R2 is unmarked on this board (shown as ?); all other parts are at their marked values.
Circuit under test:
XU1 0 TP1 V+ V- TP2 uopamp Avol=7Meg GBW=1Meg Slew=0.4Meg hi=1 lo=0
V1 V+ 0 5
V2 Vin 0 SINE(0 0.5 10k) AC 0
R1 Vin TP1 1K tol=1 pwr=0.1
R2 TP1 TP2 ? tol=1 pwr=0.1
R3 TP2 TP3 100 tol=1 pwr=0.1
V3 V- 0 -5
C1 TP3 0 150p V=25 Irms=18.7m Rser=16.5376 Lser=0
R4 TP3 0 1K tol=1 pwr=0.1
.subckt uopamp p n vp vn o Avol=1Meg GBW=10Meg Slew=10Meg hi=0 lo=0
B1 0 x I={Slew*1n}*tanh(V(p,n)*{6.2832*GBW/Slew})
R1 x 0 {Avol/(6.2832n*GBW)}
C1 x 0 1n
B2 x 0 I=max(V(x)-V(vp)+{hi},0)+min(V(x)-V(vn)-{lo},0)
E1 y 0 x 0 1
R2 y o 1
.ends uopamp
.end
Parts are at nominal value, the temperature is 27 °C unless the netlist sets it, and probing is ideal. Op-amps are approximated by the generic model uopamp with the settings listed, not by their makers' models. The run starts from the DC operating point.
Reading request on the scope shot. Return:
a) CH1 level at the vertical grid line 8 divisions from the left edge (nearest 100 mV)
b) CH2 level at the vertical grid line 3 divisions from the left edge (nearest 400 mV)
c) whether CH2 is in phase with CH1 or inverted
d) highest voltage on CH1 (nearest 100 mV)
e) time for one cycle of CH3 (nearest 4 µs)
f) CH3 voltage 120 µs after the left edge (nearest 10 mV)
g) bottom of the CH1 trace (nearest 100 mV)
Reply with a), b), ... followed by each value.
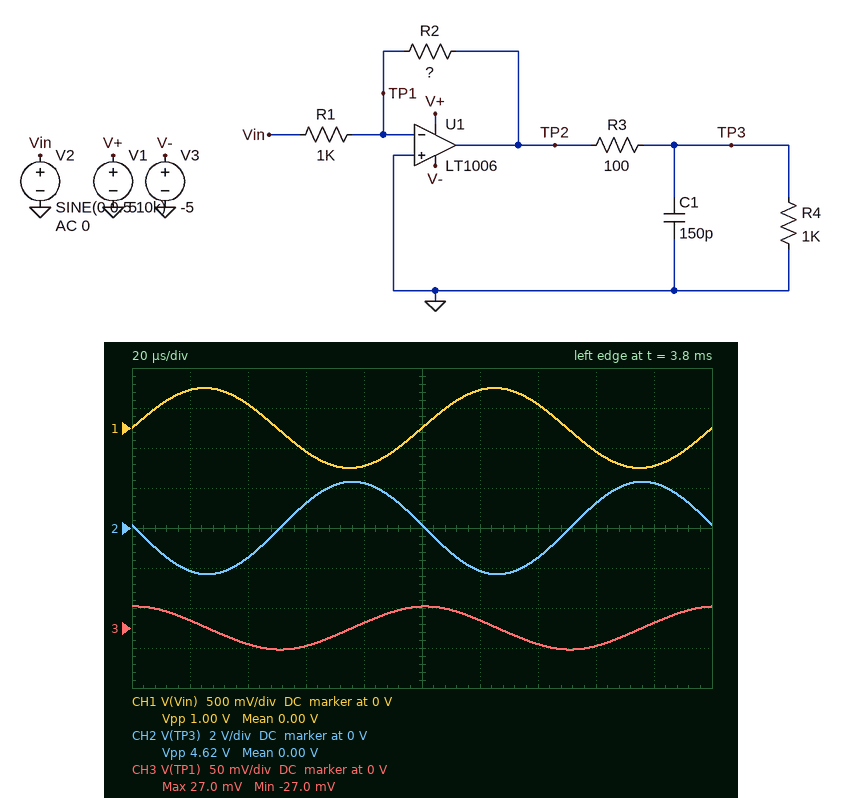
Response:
a) -300 mV
b) 1.2 V
c) inverted
d) 500 mV
e) 100 µs
f) 10 mV
g) -500 mV
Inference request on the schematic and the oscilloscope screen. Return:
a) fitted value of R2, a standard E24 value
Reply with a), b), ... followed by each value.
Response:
a) 5.1 kΩ
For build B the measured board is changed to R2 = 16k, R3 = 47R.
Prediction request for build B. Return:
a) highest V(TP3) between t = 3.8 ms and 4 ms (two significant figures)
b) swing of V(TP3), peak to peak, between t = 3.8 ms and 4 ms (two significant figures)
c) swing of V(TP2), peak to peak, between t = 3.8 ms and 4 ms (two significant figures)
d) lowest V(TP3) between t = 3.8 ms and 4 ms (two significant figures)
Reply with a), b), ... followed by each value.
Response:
a) 3.8 V
b) 8.6 V
c) 9.0 V
d) -4.8 V
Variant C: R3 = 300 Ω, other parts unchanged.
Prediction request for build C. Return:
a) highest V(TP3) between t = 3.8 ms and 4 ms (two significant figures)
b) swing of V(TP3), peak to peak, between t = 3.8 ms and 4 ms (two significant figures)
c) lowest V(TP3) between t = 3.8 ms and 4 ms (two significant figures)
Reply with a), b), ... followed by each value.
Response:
a) 2.0 V
b) 3.9 V
c) -2.0 V
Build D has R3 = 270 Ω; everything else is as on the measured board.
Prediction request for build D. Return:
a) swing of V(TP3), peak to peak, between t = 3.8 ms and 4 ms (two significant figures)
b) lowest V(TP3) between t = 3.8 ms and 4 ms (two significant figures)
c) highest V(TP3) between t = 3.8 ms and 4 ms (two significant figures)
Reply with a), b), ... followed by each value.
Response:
a) 4.0 V
b) -2.0 V
c) 2.0 V
